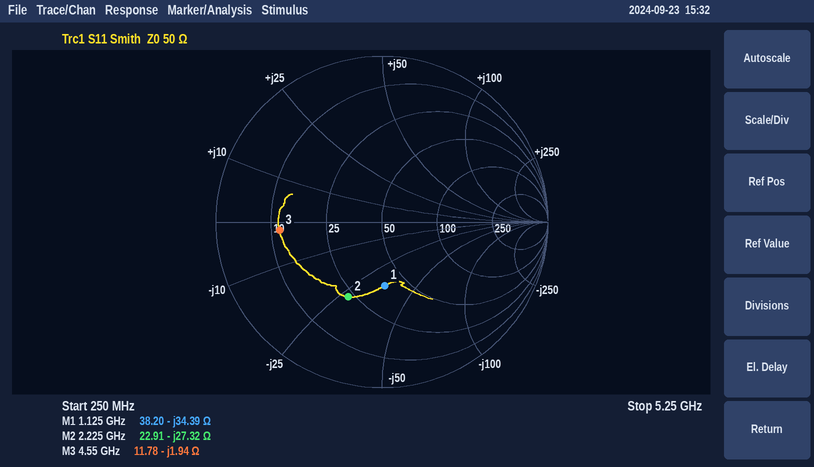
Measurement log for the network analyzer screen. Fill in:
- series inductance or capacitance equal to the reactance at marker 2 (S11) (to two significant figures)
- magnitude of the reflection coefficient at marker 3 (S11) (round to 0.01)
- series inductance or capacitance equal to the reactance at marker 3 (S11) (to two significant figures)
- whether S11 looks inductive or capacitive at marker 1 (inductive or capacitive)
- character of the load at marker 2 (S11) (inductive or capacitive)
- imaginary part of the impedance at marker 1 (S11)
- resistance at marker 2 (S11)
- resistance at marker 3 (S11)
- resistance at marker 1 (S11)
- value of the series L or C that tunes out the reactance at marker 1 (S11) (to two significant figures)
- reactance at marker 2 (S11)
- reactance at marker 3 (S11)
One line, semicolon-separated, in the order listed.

2.6 pF; 0.62; 18 pF; capacitive; capacitive; -34.39 Ω; 22.91 Ω; 11.78 Ω; 38.20 Ω; 4.9 nH; -27.32 Ω; -1.94 Ω
